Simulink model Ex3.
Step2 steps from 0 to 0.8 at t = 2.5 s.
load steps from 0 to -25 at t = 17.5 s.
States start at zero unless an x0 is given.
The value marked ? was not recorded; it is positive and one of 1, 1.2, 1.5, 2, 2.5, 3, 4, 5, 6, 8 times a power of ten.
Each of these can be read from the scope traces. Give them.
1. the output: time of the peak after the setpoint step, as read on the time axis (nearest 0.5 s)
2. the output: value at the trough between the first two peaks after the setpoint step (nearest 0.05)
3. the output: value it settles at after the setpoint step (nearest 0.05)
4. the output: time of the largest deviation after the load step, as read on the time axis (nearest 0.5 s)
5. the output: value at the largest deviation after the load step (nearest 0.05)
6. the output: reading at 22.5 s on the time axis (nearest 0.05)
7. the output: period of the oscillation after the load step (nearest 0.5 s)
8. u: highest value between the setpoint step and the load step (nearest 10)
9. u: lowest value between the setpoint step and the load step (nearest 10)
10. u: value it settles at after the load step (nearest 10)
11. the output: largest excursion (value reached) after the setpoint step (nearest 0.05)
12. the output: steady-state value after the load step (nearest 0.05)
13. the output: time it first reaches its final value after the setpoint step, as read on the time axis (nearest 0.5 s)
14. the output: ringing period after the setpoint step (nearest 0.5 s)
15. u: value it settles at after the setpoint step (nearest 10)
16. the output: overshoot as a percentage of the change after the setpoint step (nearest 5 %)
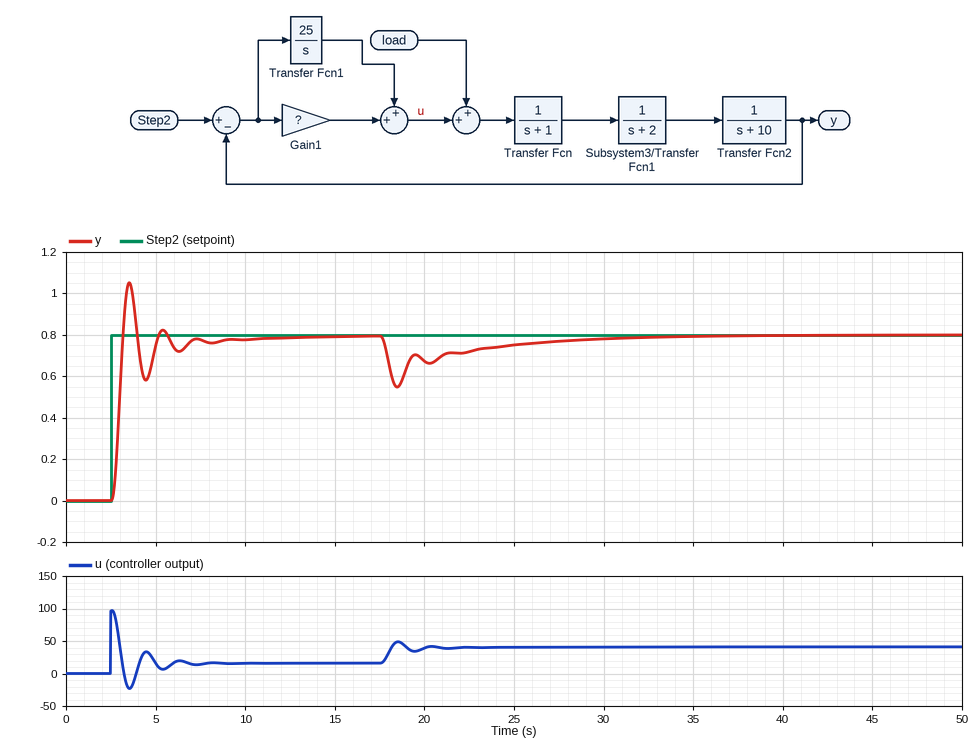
3.5 s
0.60
0.80
18.5 s
0.55
0.70
2.0 s
100
-20
40
1.05
0.80
3.0 s
2.0 s
20
30 %
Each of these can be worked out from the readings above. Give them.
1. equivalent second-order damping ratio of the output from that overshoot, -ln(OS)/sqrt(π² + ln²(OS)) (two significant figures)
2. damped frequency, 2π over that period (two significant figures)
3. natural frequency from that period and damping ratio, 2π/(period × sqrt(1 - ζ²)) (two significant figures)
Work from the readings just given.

0.36
3.1 rad/s
3.4 rad/s
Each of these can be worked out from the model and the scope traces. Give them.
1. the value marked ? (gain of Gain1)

120
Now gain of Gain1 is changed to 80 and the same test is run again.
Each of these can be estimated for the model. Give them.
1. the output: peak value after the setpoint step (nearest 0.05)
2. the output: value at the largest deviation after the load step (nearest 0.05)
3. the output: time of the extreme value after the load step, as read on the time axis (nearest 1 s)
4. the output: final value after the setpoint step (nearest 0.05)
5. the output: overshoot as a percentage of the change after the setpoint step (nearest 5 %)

0.95
0.50
19 s
0.80
20 %
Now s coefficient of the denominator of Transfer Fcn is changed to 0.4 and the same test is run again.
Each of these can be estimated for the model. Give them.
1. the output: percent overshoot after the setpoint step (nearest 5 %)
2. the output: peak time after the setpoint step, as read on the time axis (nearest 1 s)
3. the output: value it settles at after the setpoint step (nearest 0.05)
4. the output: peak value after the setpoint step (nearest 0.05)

40 %
3 s
0.80
1.10
